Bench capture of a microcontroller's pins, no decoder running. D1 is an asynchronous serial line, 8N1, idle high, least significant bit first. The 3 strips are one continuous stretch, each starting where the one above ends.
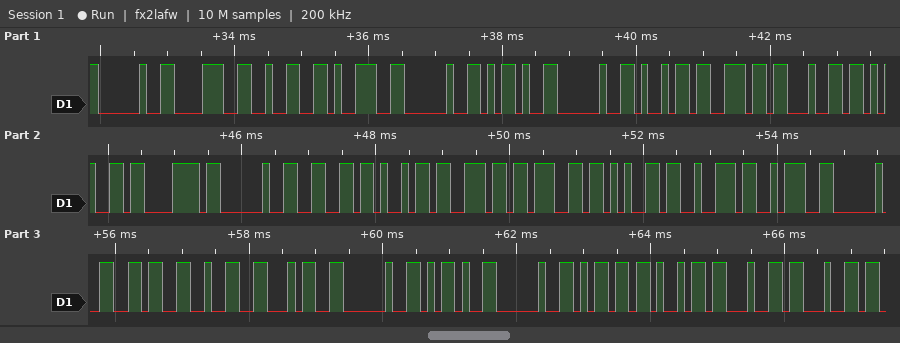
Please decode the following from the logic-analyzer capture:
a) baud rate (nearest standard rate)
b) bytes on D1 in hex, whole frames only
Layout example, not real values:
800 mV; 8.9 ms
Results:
9600 baud; 20 38 32 39 20 2D 20 69 6E 64 65 78 20 66 69 6E 67 65 72 3A 20 36 32 34 20 2D 20 6D 69 64 64
